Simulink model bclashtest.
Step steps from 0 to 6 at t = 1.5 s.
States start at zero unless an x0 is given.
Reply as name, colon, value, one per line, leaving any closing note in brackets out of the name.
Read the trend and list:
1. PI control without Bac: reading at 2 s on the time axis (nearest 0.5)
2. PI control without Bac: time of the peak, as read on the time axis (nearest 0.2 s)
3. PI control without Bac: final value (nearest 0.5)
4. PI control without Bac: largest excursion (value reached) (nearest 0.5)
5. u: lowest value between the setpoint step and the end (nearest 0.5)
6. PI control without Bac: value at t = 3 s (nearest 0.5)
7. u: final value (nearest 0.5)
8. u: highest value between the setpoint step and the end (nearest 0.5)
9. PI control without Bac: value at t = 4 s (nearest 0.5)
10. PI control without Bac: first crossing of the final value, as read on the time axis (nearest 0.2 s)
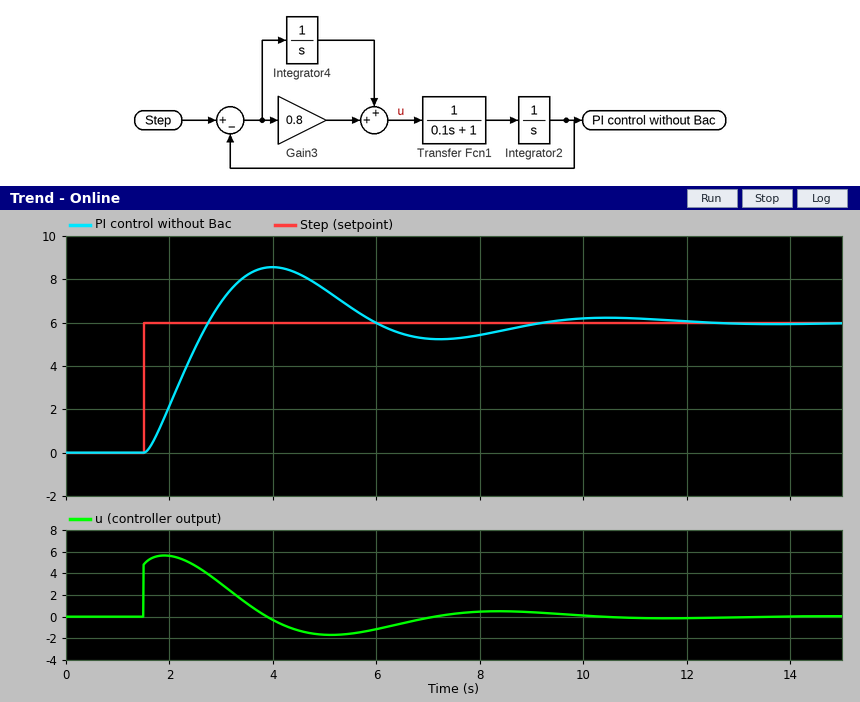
PI control without Bac: reading at 2 s on the time axis: 2.0
PI control without Bac: time of the peak, as read on the time axis: 4.0 s
PI control without Bac: final value: 6.0
PI control without Bac: largest excursion (value reached): 8.5
u: lowest value between the setpoint step and the end: -1.5
PI control without Bac: value at t = 3 s: 7.0
u: final value: 0.0
u: highest value between the setpoint step and the end: 5.5
PI control without Bac: value at t = 4 s: 8.5
PI control without Bac: first crossing of the final value, as read on the time axis: 2.8 s
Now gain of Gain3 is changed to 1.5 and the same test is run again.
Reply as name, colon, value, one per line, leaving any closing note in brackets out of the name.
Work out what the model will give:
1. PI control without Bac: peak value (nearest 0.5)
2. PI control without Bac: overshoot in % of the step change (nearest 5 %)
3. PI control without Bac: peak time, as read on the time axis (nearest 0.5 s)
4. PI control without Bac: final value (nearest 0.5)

PI control without Bac: peak value: 7.5
PI control without Bac: overshoot in % of the step change: 25 %
PI control without Bac: peak time, as read on the time axis: 3.5 s
PI control without Bac: final value: 6.0
